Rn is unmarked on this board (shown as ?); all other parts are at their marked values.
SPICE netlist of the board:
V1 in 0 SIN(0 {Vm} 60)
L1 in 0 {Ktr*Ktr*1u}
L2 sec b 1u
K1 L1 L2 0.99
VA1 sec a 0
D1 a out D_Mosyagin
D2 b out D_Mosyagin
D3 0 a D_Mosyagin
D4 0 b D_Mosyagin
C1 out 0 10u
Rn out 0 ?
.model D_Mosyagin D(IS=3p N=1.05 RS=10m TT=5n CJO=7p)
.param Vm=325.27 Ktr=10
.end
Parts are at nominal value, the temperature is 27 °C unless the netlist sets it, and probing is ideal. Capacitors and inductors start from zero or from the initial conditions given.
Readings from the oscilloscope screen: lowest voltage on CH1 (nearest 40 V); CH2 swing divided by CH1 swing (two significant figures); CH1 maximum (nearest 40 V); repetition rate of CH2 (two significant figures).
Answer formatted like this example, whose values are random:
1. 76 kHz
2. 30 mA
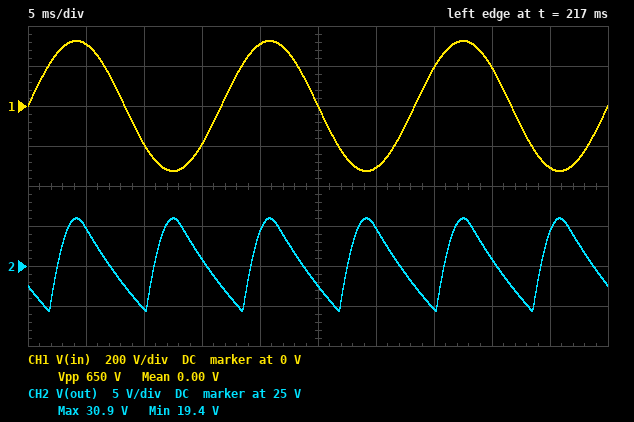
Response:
1. -320 V
2. 0.018
3. 320 V
4. 120 Hz
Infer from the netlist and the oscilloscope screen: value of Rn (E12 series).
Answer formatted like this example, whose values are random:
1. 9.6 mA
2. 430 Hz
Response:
1. 1.2 kΩ
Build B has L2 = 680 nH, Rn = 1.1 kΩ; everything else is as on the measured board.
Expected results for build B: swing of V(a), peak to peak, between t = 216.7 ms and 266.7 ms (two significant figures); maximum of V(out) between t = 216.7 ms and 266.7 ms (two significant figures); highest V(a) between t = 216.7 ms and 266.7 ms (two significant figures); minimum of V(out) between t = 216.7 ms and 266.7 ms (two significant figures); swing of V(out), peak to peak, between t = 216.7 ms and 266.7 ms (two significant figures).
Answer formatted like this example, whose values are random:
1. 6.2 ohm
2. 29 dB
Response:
1. 27 V
2. 25 V
3. 26 V
4. 15 V
5. 10 V
